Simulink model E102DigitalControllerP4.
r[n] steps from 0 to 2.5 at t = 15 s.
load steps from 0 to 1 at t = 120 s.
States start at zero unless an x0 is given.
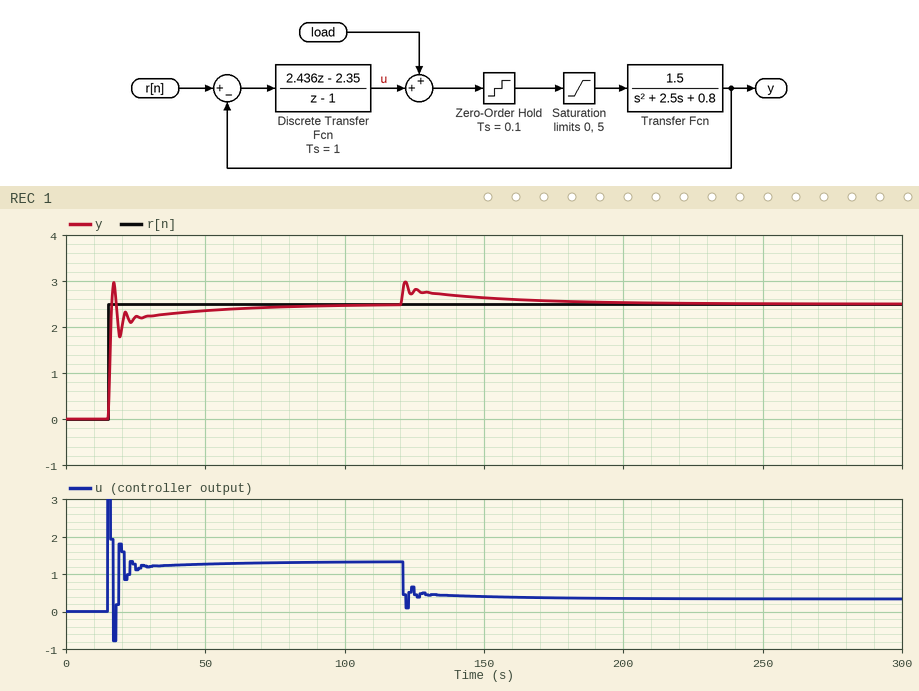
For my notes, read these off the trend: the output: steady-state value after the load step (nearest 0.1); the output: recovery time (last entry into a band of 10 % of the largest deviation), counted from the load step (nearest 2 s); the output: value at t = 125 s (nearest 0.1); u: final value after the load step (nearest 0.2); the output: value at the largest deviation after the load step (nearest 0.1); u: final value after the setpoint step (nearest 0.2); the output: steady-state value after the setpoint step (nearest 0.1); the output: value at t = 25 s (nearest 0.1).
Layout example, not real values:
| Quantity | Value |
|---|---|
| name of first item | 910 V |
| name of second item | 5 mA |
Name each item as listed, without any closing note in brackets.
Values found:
| Quantity | Value |
|---|---|
| the output: steady-state value after the load step | 2.5 |
| the output: recovery time (last entry into a band of 10 % of the largest deviation), counted from the load step | 64 s |
| the output: value at t = 125 s | 2.8 |
| u: final value after the load step | 0.4 |
| the output: value at the largest deviation after the load step | 3.0 |
| u: final value after the setpoint step | 1.4 |
| the output: steady-state value after the setpoint step | 2.5 |
| the output: value at t = 25 s | 2.2 |
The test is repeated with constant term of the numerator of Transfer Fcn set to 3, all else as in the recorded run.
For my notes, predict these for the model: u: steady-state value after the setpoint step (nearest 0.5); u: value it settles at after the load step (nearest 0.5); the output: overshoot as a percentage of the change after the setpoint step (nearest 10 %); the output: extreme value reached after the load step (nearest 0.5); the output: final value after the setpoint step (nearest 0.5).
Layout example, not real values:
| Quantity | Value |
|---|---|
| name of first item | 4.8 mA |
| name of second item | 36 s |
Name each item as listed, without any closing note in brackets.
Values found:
| Quantity | Value |
|---|---|
| u: steady-state value after the setpoint step | 0.5 |
| u: value it settles at after the load step | -0.5 |
| the output: overshoot as a percentage of the change after the setpoint step | 90 % |
| the output: extreme value reached after the load step | 3.5 |
| the output: final value after the setpoint step | 2.5 |
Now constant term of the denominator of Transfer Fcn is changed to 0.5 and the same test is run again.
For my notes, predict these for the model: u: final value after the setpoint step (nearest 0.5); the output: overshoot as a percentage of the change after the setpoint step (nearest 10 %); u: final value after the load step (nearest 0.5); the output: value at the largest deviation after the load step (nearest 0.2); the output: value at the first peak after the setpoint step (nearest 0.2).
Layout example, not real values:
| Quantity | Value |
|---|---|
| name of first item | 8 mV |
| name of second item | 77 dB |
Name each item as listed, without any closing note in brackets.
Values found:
| Quantity | Value |
|---|---|
| u: final value after the setpoint step | 1.0 |
| the output: overshoot as a percentage of the change after the setpoint step | 30 % |
| u: final value after the load step | 0.0 |
| the output: value at the largest deviation after the load step | 3.0 |
| the output: value at the first peak after the setpoint step | 3.2 |
